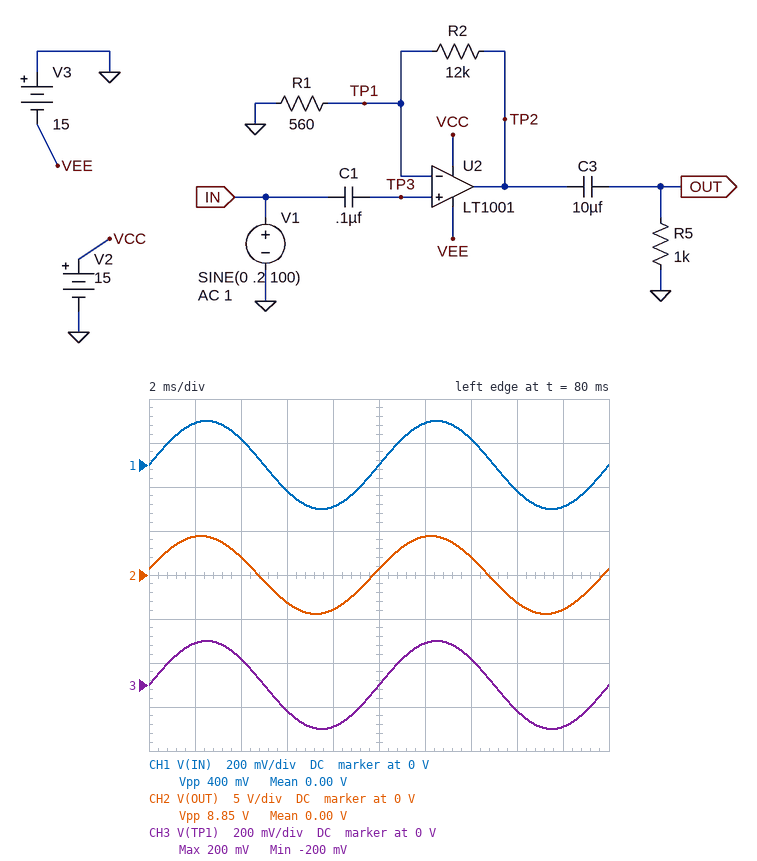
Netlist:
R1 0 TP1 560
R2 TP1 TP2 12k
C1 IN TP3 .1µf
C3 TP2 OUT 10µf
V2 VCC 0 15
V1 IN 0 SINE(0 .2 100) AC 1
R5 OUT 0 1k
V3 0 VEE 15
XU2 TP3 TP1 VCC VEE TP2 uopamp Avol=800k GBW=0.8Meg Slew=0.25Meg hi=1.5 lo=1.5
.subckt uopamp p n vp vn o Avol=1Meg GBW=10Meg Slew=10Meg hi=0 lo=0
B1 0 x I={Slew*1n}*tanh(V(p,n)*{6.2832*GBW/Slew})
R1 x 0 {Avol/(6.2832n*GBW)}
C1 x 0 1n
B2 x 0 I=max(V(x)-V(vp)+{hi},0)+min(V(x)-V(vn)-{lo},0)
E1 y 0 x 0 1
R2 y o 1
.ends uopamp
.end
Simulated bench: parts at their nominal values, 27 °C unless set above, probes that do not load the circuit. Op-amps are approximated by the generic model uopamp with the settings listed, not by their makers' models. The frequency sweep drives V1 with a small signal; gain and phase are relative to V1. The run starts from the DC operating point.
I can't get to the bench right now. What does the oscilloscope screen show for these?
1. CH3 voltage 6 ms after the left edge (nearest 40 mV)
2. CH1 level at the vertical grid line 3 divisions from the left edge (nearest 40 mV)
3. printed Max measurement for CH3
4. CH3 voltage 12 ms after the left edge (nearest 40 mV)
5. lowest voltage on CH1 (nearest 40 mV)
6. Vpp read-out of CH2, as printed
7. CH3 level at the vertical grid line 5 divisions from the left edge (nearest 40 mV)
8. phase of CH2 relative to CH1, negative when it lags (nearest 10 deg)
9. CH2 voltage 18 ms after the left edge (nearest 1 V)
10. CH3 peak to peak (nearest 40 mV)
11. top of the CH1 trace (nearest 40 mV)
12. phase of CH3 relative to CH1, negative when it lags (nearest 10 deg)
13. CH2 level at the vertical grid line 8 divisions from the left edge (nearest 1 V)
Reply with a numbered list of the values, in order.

1. -120 mV
2. -120 mV
3. 200 mV
4. 200 mV
5. -200 mV
6. 8.85 V
7. 0 V
8. 10 deg
9. -4 V
10. 400 mV
11. 200 mV
12. 0 deg
13. -3 V
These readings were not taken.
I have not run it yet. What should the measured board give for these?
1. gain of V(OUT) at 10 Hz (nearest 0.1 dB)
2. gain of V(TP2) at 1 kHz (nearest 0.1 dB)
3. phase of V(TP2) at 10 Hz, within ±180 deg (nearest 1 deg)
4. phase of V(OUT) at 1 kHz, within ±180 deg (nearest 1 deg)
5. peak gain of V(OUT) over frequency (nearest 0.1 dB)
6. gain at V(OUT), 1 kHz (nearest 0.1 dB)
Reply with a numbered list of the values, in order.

1. 21.5 dB
2. 27.0 dB
3. 0 deg
4. -1 deg
5. 27.0 dB
6. 27.0 dB
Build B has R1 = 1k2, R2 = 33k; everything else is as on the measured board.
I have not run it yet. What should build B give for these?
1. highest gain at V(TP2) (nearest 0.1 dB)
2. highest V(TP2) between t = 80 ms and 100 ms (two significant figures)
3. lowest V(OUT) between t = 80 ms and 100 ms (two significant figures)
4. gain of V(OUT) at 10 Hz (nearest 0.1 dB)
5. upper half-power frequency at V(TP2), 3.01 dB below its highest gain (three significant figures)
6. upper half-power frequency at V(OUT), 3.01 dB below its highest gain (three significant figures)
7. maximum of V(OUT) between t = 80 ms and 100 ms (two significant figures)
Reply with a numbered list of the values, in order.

1. 29.1 dB
2. 5.7 V
3. -5.6 V
4. 23.6 dB
5. 28.0 kHz
6. 28.1 kHz
7. 5.6 V
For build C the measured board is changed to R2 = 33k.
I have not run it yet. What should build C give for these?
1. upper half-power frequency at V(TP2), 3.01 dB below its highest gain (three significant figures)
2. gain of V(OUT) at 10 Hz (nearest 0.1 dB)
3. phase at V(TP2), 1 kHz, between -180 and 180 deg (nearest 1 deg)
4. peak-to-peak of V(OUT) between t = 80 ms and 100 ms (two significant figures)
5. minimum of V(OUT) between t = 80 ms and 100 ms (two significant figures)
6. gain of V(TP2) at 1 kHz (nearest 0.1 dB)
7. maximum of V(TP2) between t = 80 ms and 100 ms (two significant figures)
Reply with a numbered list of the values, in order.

1. 13.3 kHz
2. 30.1 dB
3. -4 deg
4. 24 V
5. -12 V
6. 35.5 dB
7. 12 V
